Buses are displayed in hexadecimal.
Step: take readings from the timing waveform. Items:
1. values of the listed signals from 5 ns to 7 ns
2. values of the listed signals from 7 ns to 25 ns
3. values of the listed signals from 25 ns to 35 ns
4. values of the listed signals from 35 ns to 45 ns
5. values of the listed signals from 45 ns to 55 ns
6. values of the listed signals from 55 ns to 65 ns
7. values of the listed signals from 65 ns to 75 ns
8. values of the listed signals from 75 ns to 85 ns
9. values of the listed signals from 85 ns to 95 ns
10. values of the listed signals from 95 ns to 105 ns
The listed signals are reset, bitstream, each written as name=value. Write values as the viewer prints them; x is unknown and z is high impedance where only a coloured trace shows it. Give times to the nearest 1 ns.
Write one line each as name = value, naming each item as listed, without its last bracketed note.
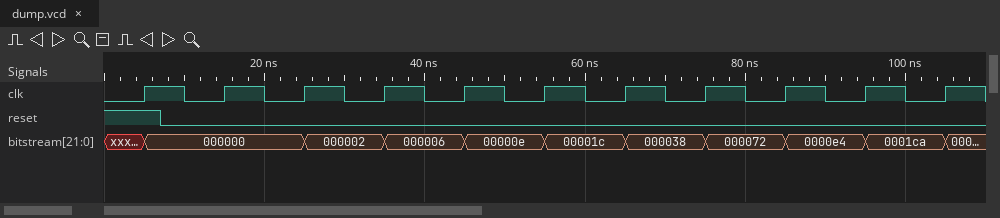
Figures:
values of the listed signals from 5 ns to 7 ns = reset=1, bitstream=000000
values of the listed signals from 7 ns to 25 ns = reset=0, bitstream=000000
values of the listed signals from 25 ns to 35 ns = reset=0, bitstream=000002
values of the listed signals from 35 ns to 45 ns = reset=0, bitstream=000006
values of the listed signals from 45 ns to 55 ns = reset=0, bitstream=00000e
values of the listed signals from 55 ns to 65 ns = reset=0, bitstream=00001c
values of the listed signals from 65 ns to 75 ns = reset=0, bitstream=000038
values of the listed signals from 75 ns to 85 ns = reset=0, bitstream=000072
values of the listed signals from 85 ns to 95 ns = reset=0, bitstream=0000e4
values of the listed signals from 95 ns to 105 ns = reset=0, bitstream=0001ca
